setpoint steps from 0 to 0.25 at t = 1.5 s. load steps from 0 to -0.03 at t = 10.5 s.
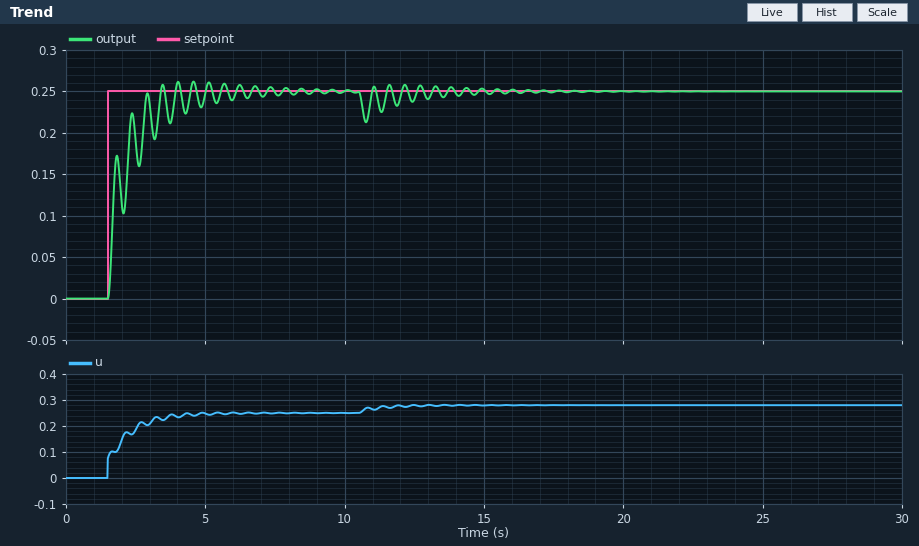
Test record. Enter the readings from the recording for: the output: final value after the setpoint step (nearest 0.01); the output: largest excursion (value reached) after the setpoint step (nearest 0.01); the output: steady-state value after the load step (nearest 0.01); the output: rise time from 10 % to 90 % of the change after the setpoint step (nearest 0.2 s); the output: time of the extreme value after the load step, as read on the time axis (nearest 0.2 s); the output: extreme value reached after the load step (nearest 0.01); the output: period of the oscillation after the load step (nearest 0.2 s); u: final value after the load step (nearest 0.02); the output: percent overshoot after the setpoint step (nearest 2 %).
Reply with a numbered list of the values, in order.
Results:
1. 0.25
2. 0.26
3. 0.25
4. 1.2 s
5. 10.8 s
6. 0.21
7. 0.6 s
8. 0.28
9. 4 %
